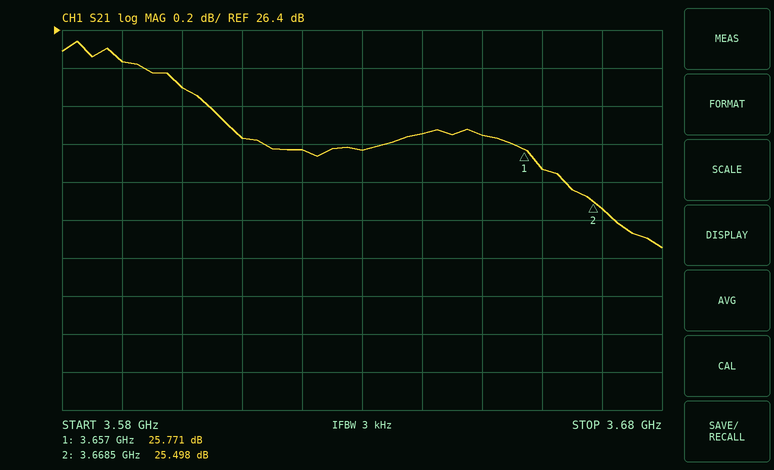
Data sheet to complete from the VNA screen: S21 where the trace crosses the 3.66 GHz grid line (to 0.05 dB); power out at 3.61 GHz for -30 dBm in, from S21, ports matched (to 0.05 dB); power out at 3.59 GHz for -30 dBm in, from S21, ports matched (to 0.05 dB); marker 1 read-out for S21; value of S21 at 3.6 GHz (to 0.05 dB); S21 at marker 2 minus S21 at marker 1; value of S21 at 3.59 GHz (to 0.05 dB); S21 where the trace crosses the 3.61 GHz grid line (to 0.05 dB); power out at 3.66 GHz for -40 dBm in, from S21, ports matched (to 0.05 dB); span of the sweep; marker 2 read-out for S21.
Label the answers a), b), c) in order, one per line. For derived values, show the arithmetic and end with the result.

a) 25.65 dB
b) -30 dBm + (25.85 dB) = -4.15 dBm
c) -30 dBm + (26.25 dB) = -3.75 dBm
d) 25.771 dB
e) 26.10 dB
f) 25.498 − (25.771) = -0.273 dB
g) 26.25 dB
h) 25.85 dB
i) -40 dBm + (25.65 dB) = -14.35 dBm
j) 100 MHz
k) 25.498 dB
